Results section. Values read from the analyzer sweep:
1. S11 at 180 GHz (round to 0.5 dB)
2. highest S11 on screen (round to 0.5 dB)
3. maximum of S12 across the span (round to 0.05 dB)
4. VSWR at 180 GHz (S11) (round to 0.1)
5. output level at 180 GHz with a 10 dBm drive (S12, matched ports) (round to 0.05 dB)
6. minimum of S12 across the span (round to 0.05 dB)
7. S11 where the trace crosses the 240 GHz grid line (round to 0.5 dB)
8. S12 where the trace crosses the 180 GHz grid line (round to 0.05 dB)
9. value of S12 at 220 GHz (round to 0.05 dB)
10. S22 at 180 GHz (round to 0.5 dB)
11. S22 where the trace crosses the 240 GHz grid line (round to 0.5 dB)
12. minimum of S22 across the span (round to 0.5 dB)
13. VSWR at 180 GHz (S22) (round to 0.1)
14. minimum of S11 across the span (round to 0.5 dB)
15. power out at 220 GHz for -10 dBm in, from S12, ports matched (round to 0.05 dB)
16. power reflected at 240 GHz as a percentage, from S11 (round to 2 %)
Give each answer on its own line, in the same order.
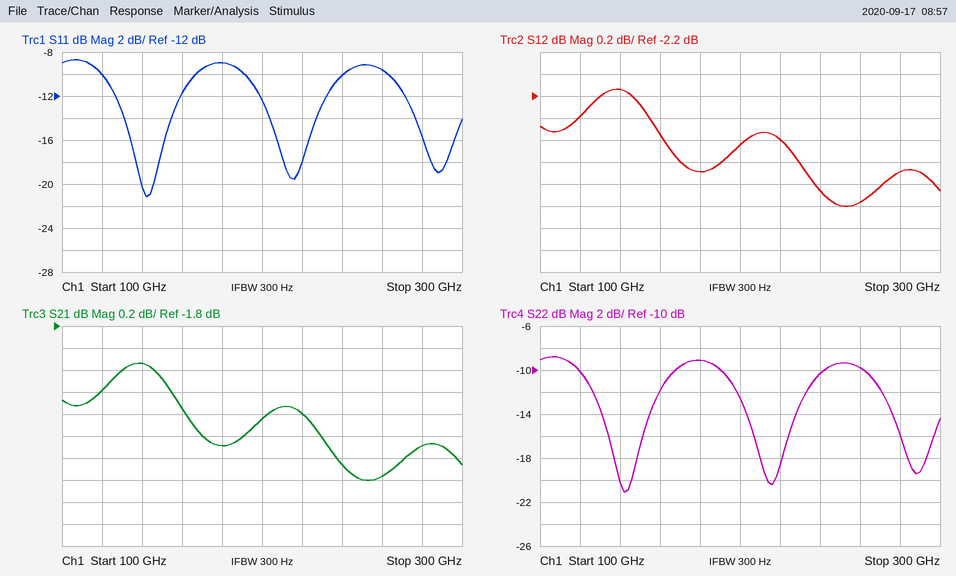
-9.0 dB
-8.5 dB
-2.15 dB
2.1
7.10 dBm
-3.20 dB
-10.0 dB
-2.90 dB
-2.60 dB
-9.0 dB
-10.5 dB
-21.0 dB
2.1
-21.0 dB
-12.60 dBm
10 %
